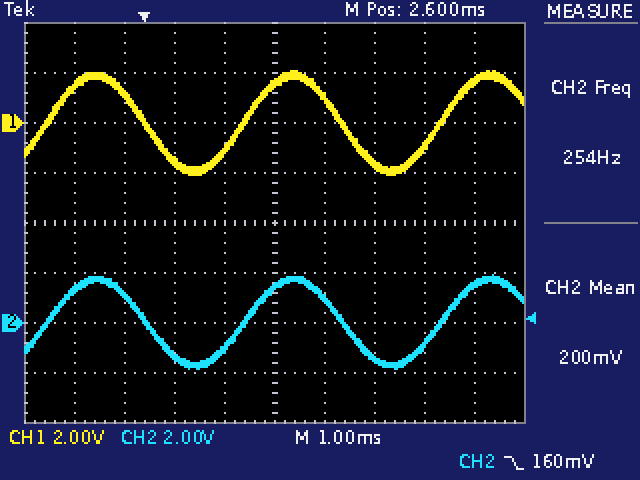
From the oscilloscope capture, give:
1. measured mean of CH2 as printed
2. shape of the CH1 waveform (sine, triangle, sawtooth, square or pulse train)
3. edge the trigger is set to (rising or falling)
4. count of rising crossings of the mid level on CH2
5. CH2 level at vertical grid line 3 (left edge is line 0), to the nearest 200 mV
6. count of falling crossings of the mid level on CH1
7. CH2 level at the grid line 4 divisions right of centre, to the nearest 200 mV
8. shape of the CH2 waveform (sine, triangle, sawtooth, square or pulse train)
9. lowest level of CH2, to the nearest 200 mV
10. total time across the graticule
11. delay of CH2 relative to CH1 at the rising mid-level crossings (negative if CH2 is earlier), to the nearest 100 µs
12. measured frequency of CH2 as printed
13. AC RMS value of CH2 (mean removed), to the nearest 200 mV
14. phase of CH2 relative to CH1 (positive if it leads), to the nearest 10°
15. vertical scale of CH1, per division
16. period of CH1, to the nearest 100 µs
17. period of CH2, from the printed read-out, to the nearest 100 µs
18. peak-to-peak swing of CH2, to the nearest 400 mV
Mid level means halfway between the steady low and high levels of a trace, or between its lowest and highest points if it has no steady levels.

200 mV
sine
falling
3
-1.4 V
2
1.6 V
sine
-1.8 V
10 ms
0.0 ms
254 Hz
1.2 V
0°
2 V
3.9 ms
3.9 ms
3.6 V
